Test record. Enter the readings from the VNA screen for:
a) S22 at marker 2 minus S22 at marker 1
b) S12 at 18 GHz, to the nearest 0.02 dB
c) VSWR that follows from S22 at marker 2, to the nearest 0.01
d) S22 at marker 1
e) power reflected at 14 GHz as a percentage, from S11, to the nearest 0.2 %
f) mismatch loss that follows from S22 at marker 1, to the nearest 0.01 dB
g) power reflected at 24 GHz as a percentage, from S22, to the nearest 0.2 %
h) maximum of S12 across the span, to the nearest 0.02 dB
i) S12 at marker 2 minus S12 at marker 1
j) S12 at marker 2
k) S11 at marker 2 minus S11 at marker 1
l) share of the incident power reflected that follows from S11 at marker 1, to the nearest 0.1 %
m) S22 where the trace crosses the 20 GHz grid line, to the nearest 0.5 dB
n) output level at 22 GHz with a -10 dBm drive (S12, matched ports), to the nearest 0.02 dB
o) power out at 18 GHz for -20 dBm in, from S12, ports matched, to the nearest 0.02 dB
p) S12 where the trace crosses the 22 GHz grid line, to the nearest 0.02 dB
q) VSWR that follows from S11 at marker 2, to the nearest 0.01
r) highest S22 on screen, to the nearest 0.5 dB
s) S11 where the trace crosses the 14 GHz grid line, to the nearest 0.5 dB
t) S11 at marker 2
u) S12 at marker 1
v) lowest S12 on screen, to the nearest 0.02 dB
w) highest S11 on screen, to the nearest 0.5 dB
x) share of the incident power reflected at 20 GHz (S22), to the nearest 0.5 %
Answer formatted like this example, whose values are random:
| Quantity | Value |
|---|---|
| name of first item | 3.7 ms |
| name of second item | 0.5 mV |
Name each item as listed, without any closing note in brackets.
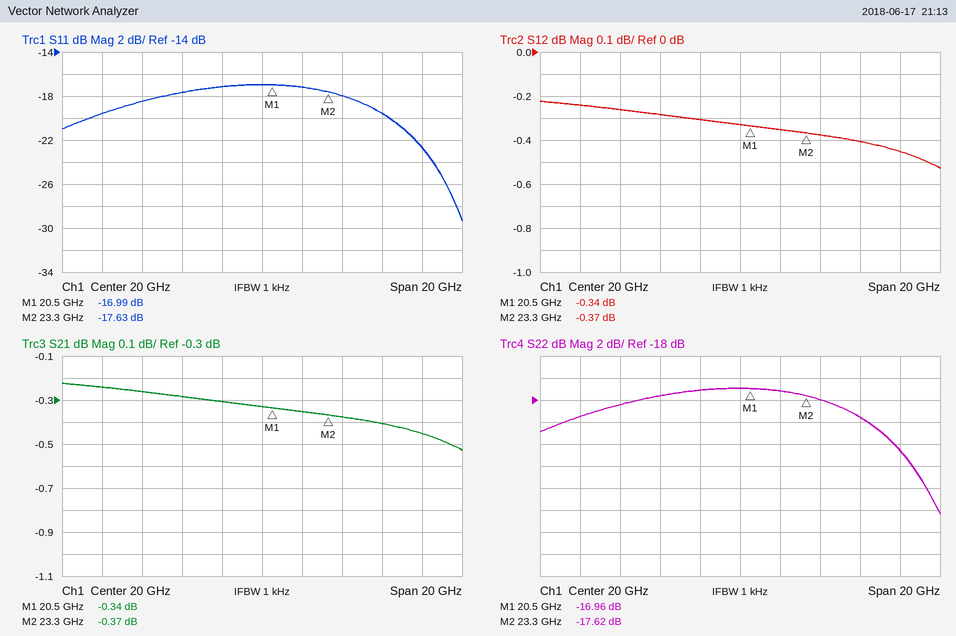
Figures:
| Quantity | Value |
|---|---|
| S22 at marker 2 minus S22 at marker 1 | -0.66 dB |
| S12 at 18 GHz, to the nearest 0.02 dB | -0.30 dB |
| VSWR that follows from S22 at marker 2, to the nearest 0.01 | 1.30 |
| S22 at marker 1 | -16.96 dB |
| power reflected at 14 GHz as a percentage, from S11, to the nearest 0.2 % | 1.4 % |
| mismatch loss that follows from S22 at marker 1, to the nearest 0.01 dB | 0.09 dB |
| power reflected at 24 GHz as a percentage, from S22, to the nearest 0.2 % | 1.6 % |
| maximum of S12 across the span, to the nearest 0.02 dB | -0.22 dB |
| S12 at marker 2 minus S12 at marker 1 | -0.03 dB |
| S12 at marker 2 | -0.37 dB |
| S11 at marker 2 minus S11 at marker 1 | -0.64 dB |
| share of the incident power reflected that follows from S11 at marker 1, to the nearest 0.1 % | 2.0 % |
| S22 where the trace crosses the 20 GHz grid line, to the nearest 0.5 dB | -17.0 dB |
| output level at 22 GHz with a -10 dBm drive (S12, matched ports), to the nearest 0.02 dB | -10.36 dBm |
| power out at 18 GHz for -20 dBm in, from S12, ports matched, to the nearest 0.02 dB | -20.30 dBm |
| S12 where the trace crosses the 22 GHz grid line, to the nearest 0.02 dB | -0.36 dB |
| VSWR that follows from S11 at marker 2, to the nearest 0.01 | 1.30 |
| highest S22 on screen, to the nearest 0.5 dB | -17.0 dB |
| S11 where the trace crosses the 14 GHz grid line, to the nearest 0.5 dB | -18.5 dB |
| S11 at marker 2 | -17.63 dB |
| S12 at marker 1 | -0.34 dB |
| lowest S12 on screen, to the nearest 0.02 dB | -0.52 dB |
| highest S11 on screen, to the nearest 0.5 dB | -17.0 dB |
| share of the incident power reflected at 20 GHz (S22), to the nearest 0.5 % | 2.0 % |
